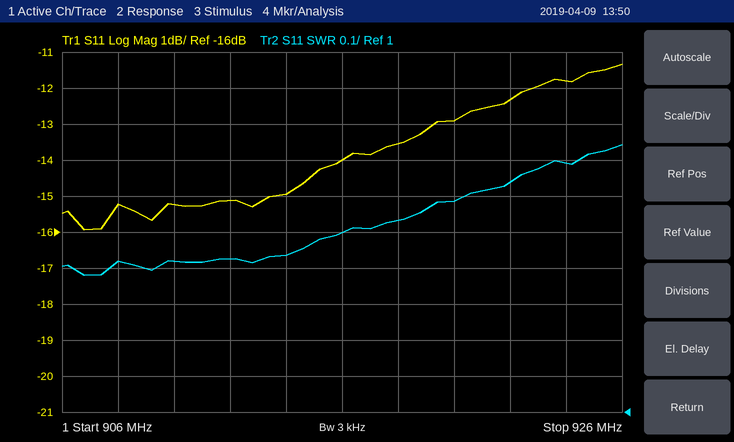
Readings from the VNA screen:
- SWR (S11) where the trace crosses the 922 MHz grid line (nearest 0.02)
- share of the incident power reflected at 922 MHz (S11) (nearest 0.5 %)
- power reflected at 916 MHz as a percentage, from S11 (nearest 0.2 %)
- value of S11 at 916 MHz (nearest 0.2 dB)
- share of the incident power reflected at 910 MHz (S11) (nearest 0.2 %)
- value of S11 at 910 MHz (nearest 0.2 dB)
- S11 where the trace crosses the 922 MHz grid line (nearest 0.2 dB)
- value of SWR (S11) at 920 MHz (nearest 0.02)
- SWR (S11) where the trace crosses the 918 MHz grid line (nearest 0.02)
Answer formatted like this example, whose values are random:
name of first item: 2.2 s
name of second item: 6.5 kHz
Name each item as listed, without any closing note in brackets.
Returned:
SWR (S11) where the trace crosses the 922 MHz grid line: 1.64
share of the incident power reflected at 922 MHz (S11): 6.0 %
power reflected at 916 MHz as a percentage, from S11: 4.0 %
value of S11 at 916 MHz: -14.0 dB
share of the incident power reflected at 910 MHz (S11): 3.0 %
value of S11 at 910 MHz: -15.2 dB
S11 where the trace crosses the 922 MHz grid line: -12.4 dB
value of SWR (S11) at 920 MHz: 1.58
SWR (S11) where the trace crosses the 918 MHz grid line: 1.54
